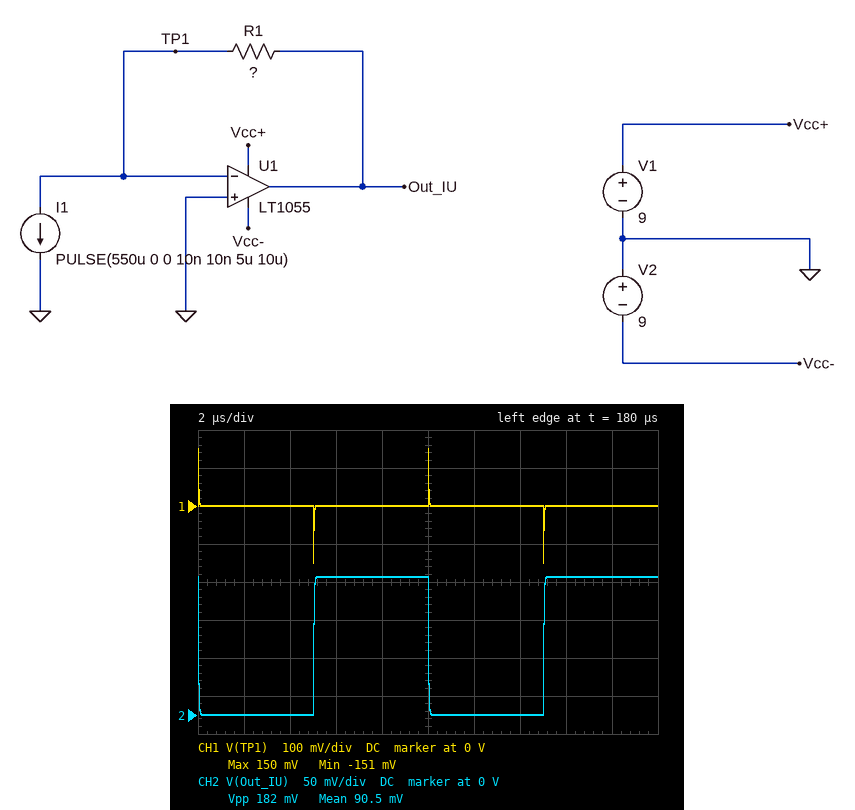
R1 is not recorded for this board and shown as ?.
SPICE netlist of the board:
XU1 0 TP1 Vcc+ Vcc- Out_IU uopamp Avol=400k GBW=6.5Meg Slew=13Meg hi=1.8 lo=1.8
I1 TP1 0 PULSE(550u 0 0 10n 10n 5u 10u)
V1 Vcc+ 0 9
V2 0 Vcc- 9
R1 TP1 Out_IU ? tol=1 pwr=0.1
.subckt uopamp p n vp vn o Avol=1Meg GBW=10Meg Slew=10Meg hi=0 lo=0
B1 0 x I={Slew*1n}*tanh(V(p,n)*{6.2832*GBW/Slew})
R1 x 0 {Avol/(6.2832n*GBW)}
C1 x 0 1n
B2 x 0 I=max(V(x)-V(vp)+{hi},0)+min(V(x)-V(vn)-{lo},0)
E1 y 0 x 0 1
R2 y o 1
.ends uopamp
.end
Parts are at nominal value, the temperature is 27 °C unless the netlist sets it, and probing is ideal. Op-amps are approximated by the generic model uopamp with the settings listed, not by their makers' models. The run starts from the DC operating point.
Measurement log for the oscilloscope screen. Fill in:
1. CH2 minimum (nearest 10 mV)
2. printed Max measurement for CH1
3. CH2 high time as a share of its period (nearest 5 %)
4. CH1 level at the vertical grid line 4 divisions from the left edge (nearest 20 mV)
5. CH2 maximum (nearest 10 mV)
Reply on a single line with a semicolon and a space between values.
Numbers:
0 V; 150 mV; 50 %; 0 V; 180 mV
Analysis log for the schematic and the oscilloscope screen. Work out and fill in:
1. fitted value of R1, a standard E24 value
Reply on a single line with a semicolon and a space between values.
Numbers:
330 Ω
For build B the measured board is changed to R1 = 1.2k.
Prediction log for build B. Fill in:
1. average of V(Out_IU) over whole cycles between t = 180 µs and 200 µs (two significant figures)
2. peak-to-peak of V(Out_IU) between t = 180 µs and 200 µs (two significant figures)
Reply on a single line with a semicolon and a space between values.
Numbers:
330 mV; 660 mV
